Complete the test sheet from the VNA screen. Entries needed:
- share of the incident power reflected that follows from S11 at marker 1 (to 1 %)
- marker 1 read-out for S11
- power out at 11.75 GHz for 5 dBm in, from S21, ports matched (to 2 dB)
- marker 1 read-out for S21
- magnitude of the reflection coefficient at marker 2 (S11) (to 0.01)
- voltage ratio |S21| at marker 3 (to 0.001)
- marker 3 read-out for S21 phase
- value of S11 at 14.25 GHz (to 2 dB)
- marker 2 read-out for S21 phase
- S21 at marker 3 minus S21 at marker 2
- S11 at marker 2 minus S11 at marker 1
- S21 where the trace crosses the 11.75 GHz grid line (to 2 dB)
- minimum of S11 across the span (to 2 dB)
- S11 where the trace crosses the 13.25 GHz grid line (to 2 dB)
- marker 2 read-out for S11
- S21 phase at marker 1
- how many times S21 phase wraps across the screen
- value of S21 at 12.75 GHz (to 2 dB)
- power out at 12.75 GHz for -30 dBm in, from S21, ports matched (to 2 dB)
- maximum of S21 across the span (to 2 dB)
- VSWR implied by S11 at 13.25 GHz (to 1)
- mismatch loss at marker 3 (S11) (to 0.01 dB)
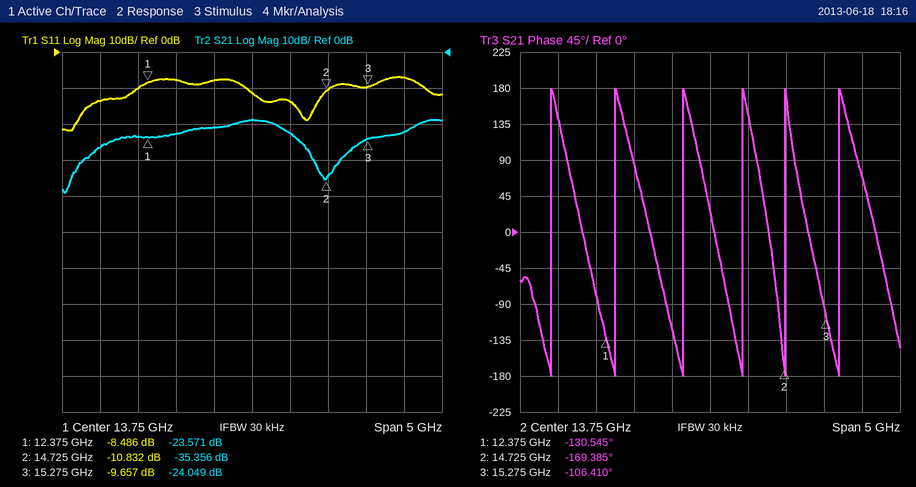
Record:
14 %
-8.486 dB
-22 dBm
-23.571 dB
0.29
0.063
-106.410°
-14 dB
-169.385°
11.307 dB
-2.346 dB
-26 dB
-22 dB
-8 dB
-10.832 dB
-130.545°
6
-22 dB
-52 dBm
-18 dB
2
0.50 dB
